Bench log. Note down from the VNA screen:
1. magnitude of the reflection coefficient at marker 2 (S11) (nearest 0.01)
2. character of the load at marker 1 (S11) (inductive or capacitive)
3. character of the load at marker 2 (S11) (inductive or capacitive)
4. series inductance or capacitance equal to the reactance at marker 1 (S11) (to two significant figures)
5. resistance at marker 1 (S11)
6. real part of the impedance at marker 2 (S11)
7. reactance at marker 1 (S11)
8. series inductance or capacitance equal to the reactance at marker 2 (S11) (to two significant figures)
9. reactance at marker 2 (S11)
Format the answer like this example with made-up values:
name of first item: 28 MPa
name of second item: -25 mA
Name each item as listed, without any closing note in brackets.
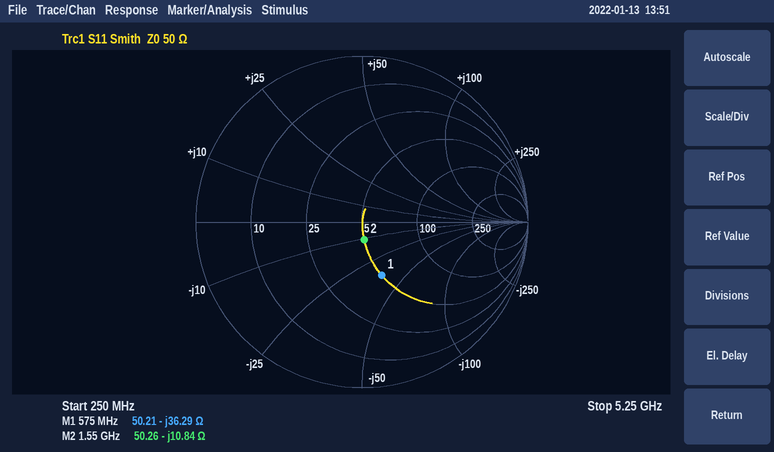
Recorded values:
magnitude of the reflection coefficient at marker 2 (S11): 0.11
character of the load at marker 1 (S11): capacitive
character of the load at marker 2 (S11): capacitive
series inductance or capacitance equal to the reactance at marker 1 (S11): 7.6 pF
resistance at marker 1: 50.21 Ω
real part of the impedance at marker 2: 50.26 Ω
reactance at marker 1: -36.29 Ω
series inductance or capacitance equal to the reactance at marker 2 (S11): 9.5 pF
reactance at marker 2: -10.84 Ω
